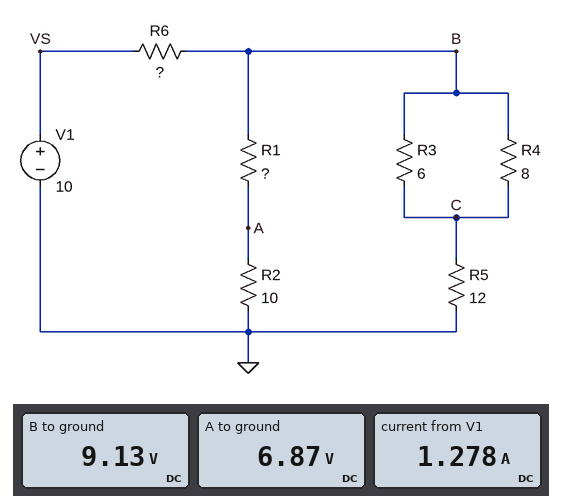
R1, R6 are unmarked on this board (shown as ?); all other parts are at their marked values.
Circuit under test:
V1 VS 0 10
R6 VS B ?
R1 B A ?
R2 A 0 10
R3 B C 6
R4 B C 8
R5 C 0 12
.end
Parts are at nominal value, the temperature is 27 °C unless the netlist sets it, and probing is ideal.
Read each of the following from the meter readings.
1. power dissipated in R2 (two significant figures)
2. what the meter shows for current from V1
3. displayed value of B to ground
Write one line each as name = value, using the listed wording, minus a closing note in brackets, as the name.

power dissipated in R2 = 4.7 W
what the meter shows for current from V1 = 1.278 A
displayed value of B to ground = 9.13 V
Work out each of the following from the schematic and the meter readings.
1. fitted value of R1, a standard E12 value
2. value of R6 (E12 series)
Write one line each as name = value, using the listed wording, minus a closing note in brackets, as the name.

fitted value of R1, a standard E12 value = 3.3 Ω
value of R6 = 0.68 Ω
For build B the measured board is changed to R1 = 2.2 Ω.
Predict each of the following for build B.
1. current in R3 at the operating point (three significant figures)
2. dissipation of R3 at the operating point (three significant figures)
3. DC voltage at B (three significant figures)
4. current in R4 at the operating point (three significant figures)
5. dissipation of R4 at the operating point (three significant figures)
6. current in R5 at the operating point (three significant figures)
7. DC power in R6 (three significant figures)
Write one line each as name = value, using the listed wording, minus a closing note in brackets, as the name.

current in R3 at the operating point = 337 mA
dissipation of R3 at the operating point = 680 mW
DC voltage at B = 9.09 V
current in R4 at the operating point = 253 mA
dissipation of R4 at the operating point = 510 mW
current in R5 at the operating point = 589 mA
DC power in R6 = 1.21 W
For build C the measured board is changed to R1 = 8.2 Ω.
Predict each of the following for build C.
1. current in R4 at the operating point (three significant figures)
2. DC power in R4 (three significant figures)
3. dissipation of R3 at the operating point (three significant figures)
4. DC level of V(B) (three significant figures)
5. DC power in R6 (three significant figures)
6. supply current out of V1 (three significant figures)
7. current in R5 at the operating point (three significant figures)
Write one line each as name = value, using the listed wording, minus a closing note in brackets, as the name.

current in R4 at the operating point = 257 mA
DC power in R4 = 528 mW
dissipation of R3 at the operating point = 704 mW
DC level of V(B) = 9.25 V
DC power in R6 = 834 mW
supply current out of V1 = 1.11 A
current in R5 at the operating point = 599 mA
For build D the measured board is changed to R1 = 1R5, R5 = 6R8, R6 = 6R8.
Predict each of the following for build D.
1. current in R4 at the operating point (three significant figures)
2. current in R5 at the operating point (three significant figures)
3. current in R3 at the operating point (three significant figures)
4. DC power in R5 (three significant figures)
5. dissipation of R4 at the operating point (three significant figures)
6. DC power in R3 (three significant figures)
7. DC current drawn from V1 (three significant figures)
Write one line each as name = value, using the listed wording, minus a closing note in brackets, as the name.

current in R4 at the operating point = 186 mA
current in R5 at the operating point = 433 mA
current in R3 at the operating point = 248 mA
DC power in R5 = 1.28 W
dissipation of R4 at the operating point = 276 mW
DC power in R3 = 368 mW
DC current drawn from V1 = 819 mA
